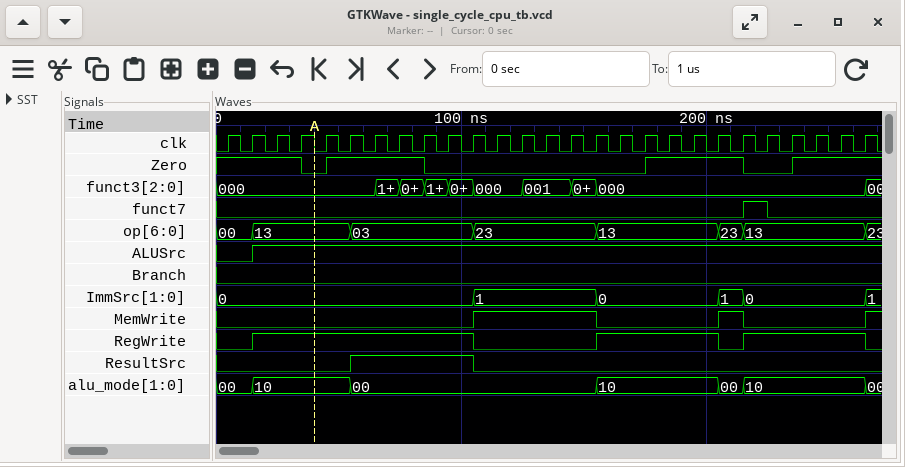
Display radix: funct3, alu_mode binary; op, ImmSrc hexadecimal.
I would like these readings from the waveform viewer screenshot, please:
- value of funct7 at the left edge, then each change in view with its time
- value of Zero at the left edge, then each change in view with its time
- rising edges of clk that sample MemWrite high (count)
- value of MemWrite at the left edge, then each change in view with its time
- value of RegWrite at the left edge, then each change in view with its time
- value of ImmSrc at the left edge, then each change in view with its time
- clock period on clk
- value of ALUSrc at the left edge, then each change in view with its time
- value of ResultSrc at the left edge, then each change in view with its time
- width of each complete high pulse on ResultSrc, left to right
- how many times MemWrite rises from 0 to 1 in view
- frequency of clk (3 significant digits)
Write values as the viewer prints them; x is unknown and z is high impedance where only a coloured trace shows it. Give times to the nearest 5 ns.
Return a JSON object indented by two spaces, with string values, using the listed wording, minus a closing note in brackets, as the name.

{
  "value of funct7 at the left edge, then each change in view with its time": "0, 1 at 215 ns, 0 at 225 ns",
  "value of Zero at the left edge, then each change in view with its time": "1, 0 at 35 ns, 1 at 45 ns, 0 at 85 ns, 1 at 175 ns, 0 at 215 ns, 1 at 235 ns",
  "rising edges of clk that sample MemWrite high": "6",
  "value of MemWrite at the left edge, then each change in view with its time": "0, 1 at 105 ns, 0 at 155 ns, 1 at 205 ns, 0 at 215 ns, 1 at 265 ns",
  "value of RegWrite at the left edge, then each change in view with its time": "0, 1 at 15 ns, 0 at 105 ns, 1 at 155 ns, 0 at 205 ns, 1 at 215 ns, 0 at 265 ns",
  "value of ImmSrc at the left edge, then each change in view with its time": "0, 1 at 105 ns, 0 at 155 ns, 1 at 205 ns, 0 at 215 ns, 1 at 265 ns",
  "clock period on clk": "10 ns",
  "value of ALUSrc at the left edge, then each change in view with its time": "0, 1 at 15 ns",
  "value of ResultSrc at the left edge, then each change in view with its time": "0, 1 at 55 ns, 0 at 105 ns",
  "width of each complete high pulse on ResultSrc, left to right": "50 ns",
  "how many times MemWrite rises from 0 to 1 in view": "3",
  "frequency of clk": "100 MHz"
}
